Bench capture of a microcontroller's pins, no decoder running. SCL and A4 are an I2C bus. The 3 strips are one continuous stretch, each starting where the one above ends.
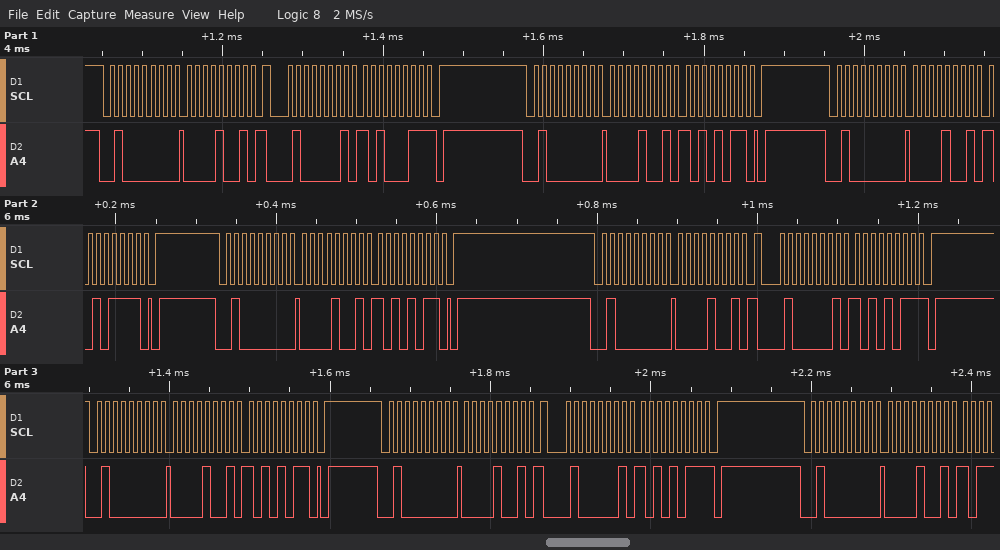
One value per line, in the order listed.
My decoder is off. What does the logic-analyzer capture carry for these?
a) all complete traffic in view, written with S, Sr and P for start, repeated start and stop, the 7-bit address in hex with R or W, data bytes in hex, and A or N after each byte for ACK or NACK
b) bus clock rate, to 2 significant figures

S 20W A 09 A Sr 20R A A3 N P S 20W A 09 A AB A P S 20W A 09 A AF A P S 20W A 09 A AB A P S 20W A 09 A Sr 20R A AB N P S 20W A 09 A AB A P S 20W A 09 A Sr 20R A AB N P S 20W A 09 A
100 kHz
